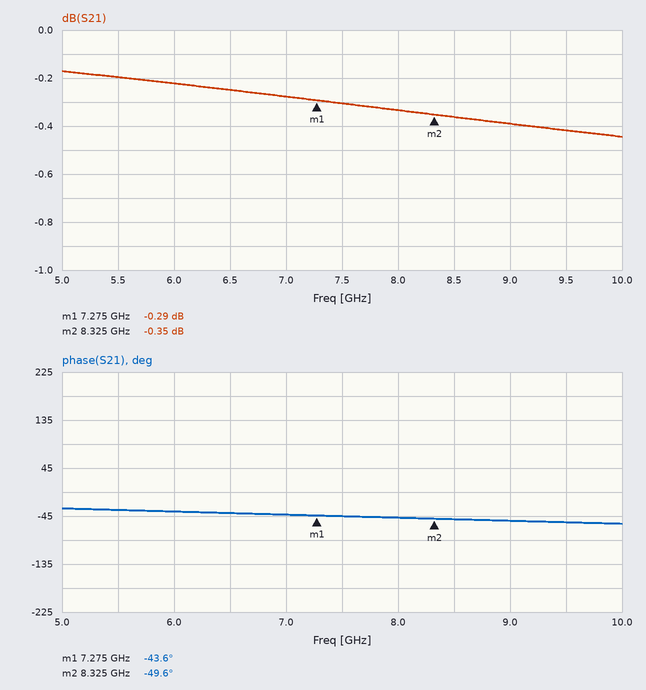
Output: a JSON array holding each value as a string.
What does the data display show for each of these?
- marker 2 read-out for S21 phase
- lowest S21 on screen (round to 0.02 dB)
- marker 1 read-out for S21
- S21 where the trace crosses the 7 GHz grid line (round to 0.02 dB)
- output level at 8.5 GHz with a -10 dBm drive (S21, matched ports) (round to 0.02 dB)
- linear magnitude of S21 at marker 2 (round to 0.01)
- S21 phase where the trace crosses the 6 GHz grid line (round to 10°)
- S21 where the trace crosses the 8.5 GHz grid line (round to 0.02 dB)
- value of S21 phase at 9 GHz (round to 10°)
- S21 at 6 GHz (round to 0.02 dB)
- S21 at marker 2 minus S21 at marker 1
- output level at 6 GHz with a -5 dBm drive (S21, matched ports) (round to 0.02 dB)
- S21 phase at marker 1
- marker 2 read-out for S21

["-49.6°", "-0.44 dB", "-0.29 dB", "-0.28 dB", "-10.36 dBm", "0.96", "-40°", "-0.36 dB", "-50°", "-0.22 dB", "-0.06 dB", "-5.22 dBm", "-43.6°", "-0.35 dB"]
